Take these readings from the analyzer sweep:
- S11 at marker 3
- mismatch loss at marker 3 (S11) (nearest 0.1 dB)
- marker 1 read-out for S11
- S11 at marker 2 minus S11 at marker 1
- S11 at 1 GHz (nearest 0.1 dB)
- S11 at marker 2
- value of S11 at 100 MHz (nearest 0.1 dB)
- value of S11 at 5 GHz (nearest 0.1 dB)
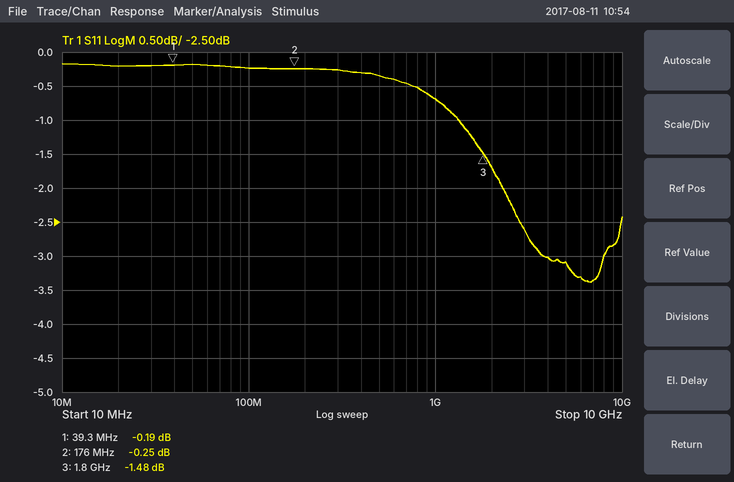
-1.48 dB
5.4 dB
-0.19 dB
-0.06 dB
-0.7 dB
-0.25 dB
-0.2 dB
-3.1 dB
